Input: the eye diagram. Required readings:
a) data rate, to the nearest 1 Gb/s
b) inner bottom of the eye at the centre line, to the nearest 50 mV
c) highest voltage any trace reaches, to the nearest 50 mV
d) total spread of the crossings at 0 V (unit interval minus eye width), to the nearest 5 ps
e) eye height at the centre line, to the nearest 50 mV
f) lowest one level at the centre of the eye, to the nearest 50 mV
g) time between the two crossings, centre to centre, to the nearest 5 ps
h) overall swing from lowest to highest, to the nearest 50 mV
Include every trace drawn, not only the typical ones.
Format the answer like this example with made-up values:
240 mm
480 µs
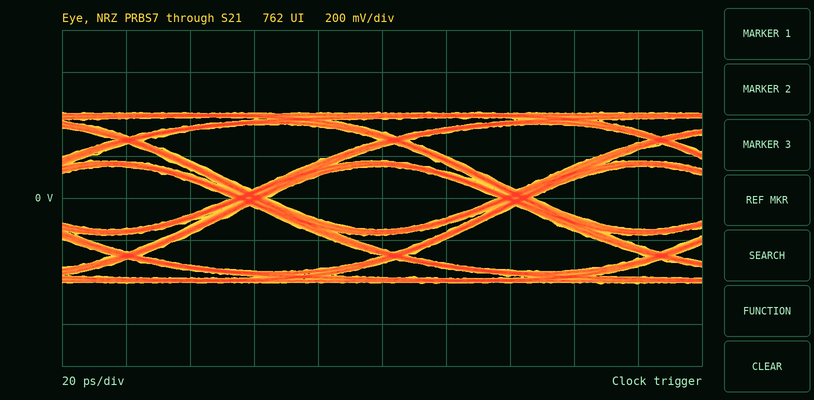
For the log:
12 Gb/s
-150 mV
400 mV
10 ps
300 mV
150 mV
85 ps
800 mV
